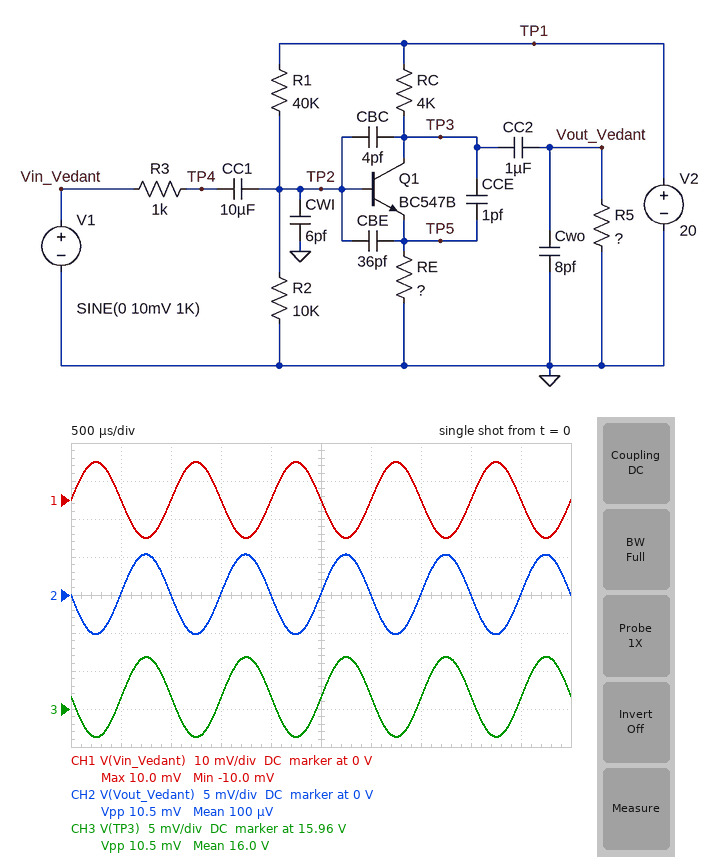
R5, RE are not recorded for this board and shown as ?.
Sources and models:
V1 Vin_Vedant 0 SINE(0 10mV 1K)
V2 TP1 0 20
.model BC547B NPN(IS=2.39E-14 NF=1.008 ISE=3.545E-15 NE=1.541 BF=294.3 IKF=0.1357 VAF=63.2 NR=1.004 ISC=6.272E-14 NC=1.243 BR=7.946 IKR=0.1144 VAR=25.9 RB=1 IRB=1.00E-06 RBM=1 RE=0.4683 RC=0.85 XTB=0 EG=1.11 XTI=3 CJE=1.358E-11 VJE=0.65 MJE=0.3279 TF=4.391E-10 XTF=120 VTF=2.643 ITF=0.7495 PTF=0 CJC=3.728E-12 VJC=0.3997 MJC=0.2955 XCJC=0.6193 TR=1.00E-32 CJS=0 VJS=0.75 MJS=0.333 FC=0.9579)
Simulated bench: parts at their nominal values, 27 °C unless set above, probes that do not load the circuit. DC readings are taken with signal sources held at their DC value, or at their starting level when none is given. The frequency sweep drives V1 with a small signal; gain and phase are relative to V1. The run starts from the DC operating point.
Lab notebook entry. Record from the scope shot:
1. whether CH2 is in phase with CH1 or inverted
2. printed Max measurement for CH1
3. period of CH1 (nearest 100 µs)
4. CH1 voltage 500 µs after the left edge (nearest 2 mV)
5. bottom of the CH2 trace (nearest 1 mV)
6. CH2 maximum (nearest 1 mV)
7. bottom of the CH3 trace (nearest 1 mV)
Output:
inverted
10.0 mV
1.0 ms
0 V
-5 mV
5 mV
15.956 V
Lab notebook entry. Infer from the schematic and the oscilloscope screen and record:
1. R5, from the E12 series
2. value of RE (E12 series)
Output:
3.9 kΩ
3.3 kΩ
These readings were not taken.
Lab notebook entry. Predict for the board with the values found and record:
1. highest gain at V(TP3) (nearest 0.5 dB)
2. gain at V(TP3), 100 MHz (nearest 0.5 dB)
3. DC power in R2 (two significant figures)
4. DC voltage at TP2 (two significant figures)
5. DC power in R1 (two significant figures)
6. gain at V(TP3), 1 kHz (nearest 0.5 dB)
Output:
0 dB
-23.0 dB
1.6 mW
4.0 V
6.4 mW
-5.5 dB
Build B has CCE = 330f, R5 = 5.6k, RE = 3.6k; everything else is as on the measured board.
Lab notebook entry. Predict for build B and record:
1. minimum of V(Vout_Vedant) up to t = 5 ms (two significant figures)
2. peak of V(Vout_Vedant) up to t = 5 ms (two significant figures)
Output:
-5.6 mV
5.8 mV
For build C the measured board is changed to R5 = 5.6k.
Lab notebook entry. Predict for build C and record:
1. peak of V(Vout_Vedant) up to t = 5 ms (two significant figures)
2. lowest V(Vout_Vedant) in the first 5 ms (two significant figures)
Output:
6.3 mV
-6.1 mV
